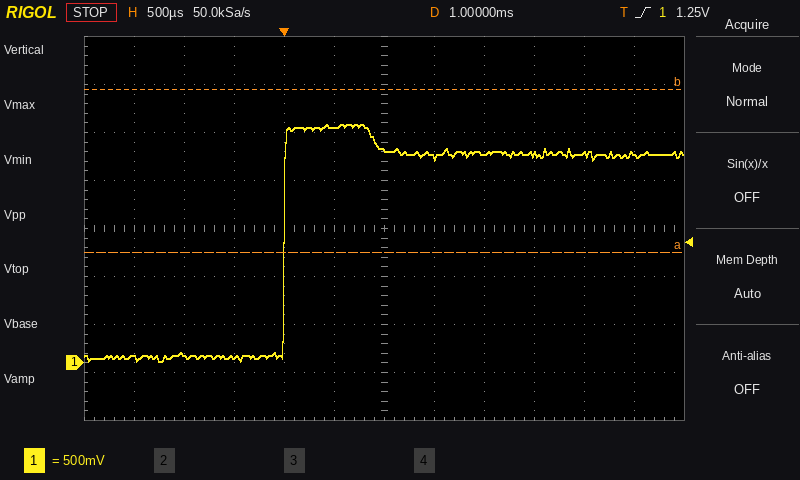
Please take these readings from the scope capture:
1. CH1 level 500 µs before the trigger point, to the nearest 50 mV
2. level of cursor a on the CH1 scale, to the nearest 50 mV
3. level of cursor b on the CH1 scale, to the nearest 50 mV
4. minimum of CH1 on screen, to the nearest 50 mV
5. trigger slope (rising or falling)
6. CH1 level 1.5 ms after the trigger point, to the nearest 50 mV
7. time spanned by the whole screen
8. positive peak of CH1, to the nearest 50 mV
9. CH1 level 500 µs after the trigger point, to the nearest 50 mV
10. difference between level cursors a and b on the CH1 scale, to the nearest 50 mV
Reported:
50 mV
1.15 V
2.85 V
0 mV
rising
2.15 V
6 ms
2.50 V
2.45 V
1.70 V
